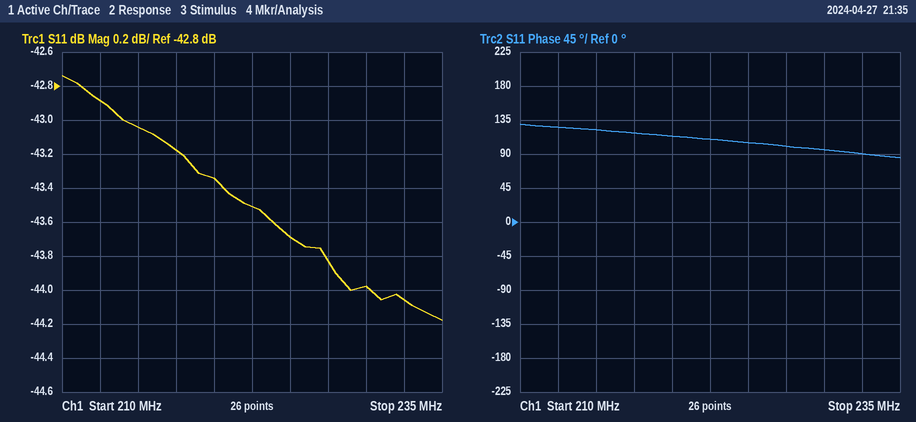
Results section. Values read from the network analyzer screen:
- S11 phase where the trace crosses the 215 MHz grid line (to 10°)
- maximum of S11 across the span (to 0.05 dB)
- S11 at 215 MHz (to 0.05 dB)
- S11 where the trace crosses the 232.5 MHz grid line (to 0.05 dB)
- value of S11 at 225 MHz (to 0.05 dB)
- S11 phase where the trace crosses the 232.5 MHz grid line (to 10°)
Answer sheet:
120°
-42.75 dB
-43.05 dB
-44.05 dB
-43.70 dB
90°
